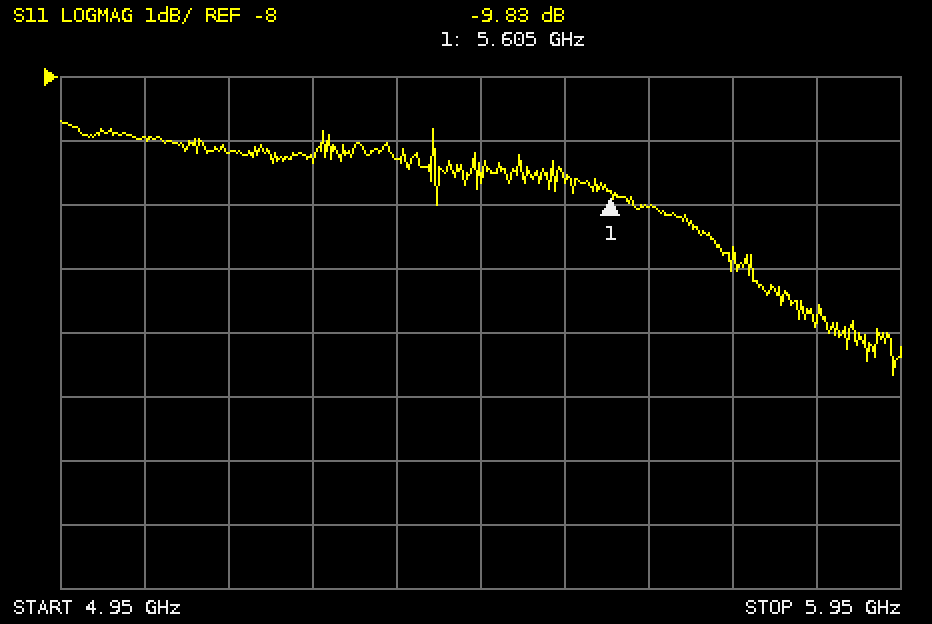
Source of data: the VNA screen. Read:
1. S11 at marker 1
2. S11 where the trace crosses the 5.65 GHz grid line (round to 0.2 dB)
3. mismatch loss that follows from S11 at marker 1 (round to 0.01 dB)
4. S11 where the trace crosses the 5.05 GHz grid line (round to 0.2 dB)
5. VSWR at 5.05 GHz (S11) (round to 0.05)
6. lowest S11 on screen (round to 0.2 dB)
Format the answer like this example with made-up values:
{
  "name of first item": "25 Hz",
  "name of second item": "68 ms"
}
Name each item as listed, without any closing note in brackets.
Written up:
{
  "S11 at marker 1": "-9.83 dB",
  "S11 where the trace crosses the 5.65 GHz grid line": "-10.0 dB",
  "mismatch loss that follows from S11 at marker 1": "0.48 dB",
  "S11 where the trace crosses the 5.05 GHz grid line": "-9.0 dB",
  "VSWR at 5.05 GHz (S11)": "2.10",
  "lowest S11 on screen": "-12.6 dB"
}
